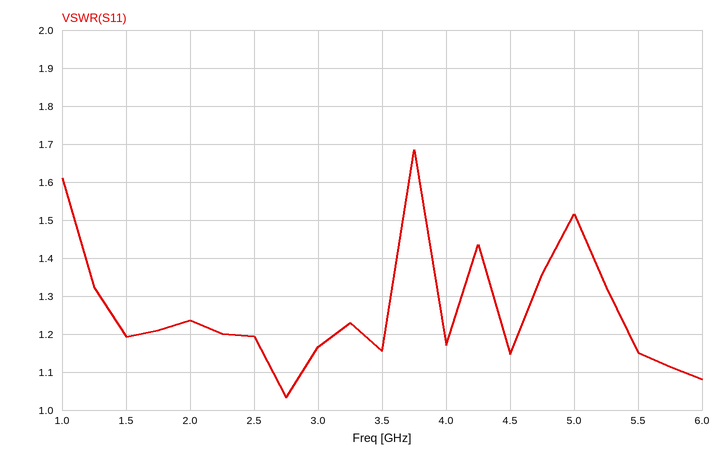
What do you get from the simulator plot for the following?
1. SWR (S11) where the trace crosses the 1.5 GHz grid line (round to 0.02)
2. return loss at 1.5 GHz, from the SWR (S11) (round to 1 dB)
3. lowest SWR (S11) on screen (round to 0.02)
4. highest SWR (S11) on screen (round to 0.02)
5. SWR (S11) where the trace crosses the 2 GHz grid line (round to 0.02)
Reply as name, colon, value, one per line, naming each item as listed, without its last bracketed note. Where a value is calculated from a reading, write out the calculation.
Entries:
SWR (S11) where the trace crosses the 1.5 GHz grid line: 1.20
return loss at 1.5 GHz, from the SWR (S11): −20 log10((1.2 − 1)/(1.2 + 1)) ≈ 21 dB
lowest SWR (S11) on screen: 1.04
highest SWR (S11) on screen: 1.68
SWR (S11) where the trace crosses the 2 GHz grid line: 1.24
